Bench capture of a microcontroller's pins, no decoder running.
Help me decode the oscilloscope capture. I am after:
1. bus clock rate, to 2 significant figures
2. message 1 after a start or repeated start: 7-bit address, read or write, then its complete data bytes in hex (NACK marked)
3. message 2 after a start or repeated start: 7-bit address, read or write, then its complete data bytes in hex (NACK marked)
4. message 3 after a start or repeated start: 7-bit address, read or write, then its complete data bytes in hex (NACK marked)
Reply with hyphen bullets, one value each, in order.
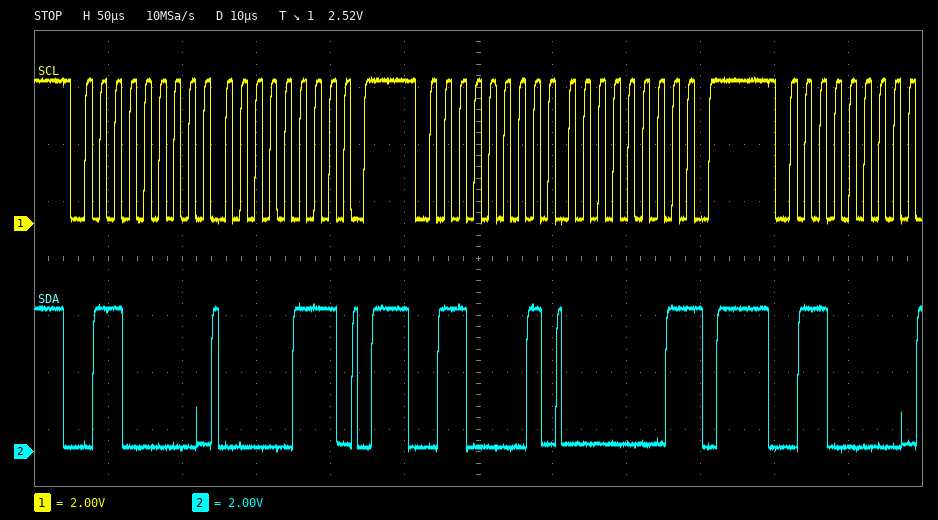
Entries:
- 100 kHz
- 0x30 write: 07
- 0x30 read: 01 NACK
- 0x30 write
